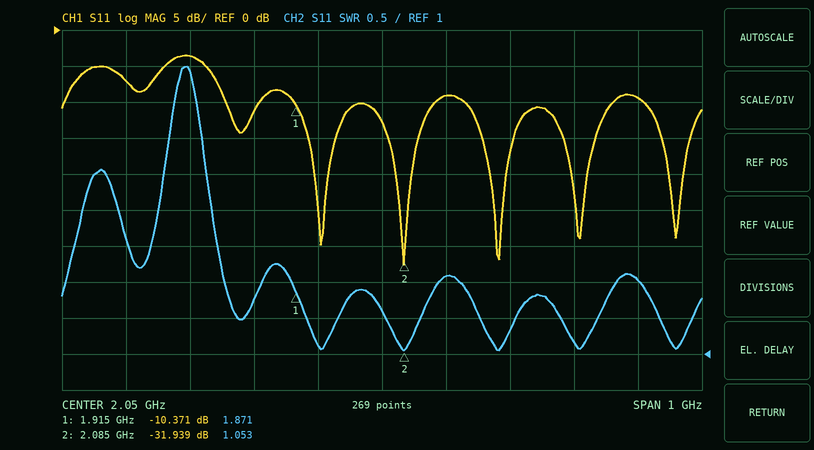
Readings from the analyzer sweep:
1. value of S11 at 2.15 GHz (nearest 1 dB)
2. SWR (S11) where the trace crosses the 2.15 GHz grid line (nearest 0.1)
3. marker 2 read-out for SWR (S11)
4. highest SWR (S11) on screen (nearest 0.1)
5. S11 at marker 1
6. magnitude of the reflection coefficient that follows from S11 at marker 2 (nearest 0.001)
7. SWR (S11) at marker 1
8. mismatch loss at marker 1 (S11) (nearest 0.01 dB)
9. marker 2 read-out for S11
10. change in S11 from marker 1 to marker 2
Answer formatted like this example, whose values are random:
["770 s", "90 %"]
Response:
["-9 dB", "2.1", "1.053", "5.0", "-10.371 dB", "0.025", "1.871", "0.42 dB", "-31.939 dB", "-21.568 dB"]
